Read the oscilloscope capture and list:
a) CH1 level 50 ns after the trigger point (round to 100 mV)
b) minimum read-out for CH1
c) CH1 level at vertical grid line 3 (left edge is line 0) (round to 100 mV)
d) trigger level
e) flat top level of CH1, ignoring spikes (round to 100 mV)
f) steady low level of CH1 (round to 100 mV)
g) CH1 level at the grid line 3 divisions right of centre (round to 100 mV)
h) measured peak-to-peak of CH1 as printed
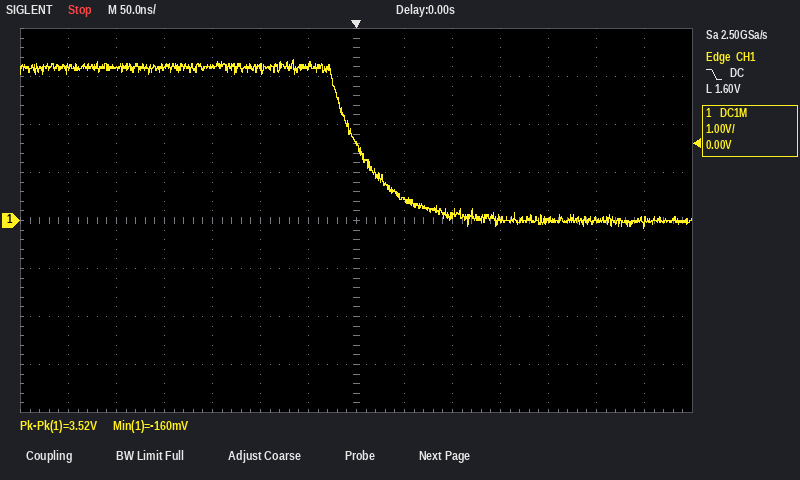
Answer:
400 mV
-160 mV
3.2 V
1.60 V
3.2 V
0.0 V
0.0 V
3.52 V
